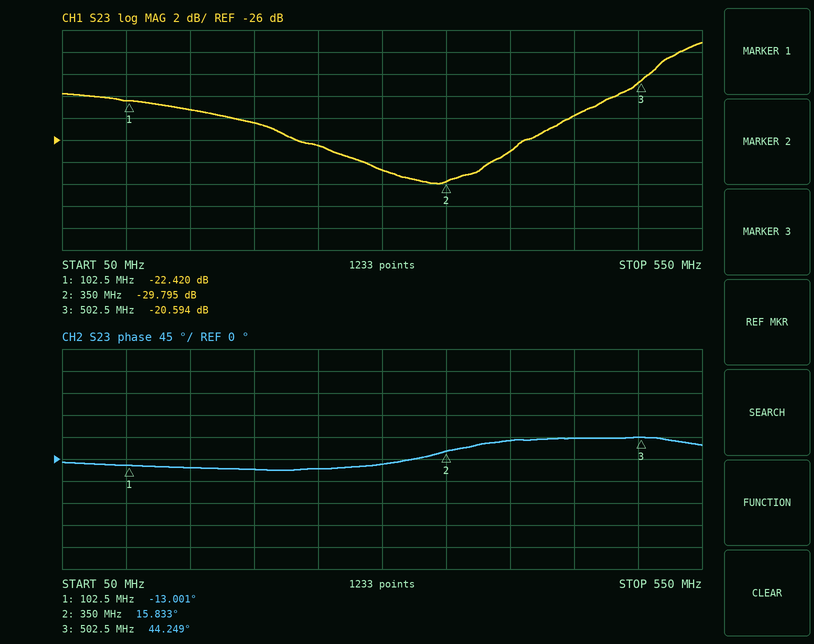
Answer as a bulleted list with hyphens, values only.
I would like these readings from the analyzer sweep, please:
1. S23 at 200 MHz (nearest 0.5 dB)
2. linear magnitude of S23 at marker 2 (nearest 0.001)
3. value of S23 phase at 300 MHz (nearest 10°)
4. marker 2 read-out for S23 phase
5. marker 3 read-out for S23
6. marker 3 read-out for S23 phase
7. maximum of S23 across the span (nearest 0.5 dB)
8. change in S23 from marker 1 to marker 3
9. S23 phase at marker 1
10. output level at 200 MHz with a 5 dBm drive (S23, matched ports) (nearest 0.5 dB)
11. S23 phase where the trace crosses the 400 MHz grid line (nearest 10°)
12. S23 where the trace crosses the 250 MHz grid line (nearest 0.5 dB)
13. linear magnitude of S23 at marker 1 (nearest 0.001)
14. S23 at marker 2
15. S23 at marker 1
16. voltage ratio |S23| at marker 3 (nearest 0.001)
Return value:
- -24.5 dB
- 0.032
- -10°
- 15.833°
- -20.594 dB
- 44.249°
- -17.0 dB
- 1.826 dB
- -13.001°
- -19.5 dBm
- 40°
- -26.5 dB
- 0.076
- -29.795 dB
- -22.420 dB
- 0.093
